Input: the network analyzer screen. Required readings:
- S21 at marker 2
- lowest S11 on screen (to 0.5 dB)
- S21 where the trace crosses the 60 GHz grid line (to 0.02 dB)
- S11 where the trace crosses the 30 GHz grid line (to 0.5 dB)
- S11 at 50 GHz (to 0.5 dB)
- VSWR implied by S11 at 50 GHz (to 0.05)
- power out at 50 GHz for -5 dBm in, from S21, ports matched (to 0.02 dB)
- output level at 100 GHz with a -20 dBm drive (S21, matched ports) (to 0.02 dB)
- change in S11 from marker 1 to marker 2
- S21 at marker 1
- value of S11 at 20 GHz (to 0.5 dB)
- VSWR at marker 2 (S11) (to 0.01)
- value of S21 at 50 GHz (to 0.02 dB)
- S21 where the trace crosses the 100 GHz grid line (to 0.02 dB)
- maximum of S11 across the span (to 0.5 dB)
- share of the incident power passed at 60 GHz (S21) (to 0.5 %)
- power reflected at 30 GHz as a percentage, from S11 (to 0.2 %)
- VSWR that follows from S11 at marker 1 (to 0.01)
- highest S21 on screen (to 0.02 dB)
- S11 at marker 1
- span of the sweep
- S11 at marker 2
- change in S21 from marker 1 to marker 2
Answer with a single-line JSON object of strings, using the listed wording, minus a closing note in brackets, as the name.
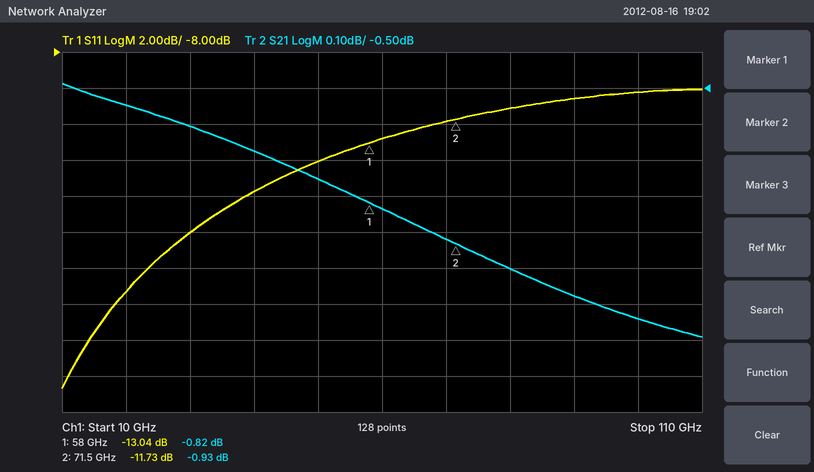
{"S21 at marker 2": "-0.93 dB", "lowest S11 on screen": "-26.5 dB", "S21 where the trace crosses the 60 GHz grid line": "-0.84 dB", "S11 where the trace crosses the 30 GHz grid line": "-18.0 dB", "S11 at 50 GHz": "-14.0 dB", "VSWR implied by S11 at 50 GHz": "1.50", "power out at 50 GHz for -5 dBm in, from S21, ports matched": "-5.76 dBm", "output level at 100 GHz with a -20 dBm drive (S21, matched ports)": "-21.14 dBm", "change in S11 from marker 1 to marker 2": "1.31 dB", "S21 at marker 1": "-0.82 dB", "value of S11 at 20 GHz": "-21.5 dB", "VSWR at marker 2 (S11)": "1.70", "value of S21 at 50 GHz": "-0.76 dB", "S21 where the trace crosses the 100 GHz grid line": "-1.14 dB", "maximum of S11 across the span": "-10.0 dB", "share of the incident power passed at 60 GHz (S21)": "82.5 %", "power reflected at 30 GHz as a percentage, from S11": "1.6 %", "VSWR that follows from S11 at marker 1": "1.57", "highest S21 on screen": "-0.48 dB", "S11 at marker 1": "-13.04 dB", "span of the sweep": "100 GHz", "S11 at marker 2": "-11.73 dB", "change in S21 from marker 1 to marker 2": "-0.11 dB"}
